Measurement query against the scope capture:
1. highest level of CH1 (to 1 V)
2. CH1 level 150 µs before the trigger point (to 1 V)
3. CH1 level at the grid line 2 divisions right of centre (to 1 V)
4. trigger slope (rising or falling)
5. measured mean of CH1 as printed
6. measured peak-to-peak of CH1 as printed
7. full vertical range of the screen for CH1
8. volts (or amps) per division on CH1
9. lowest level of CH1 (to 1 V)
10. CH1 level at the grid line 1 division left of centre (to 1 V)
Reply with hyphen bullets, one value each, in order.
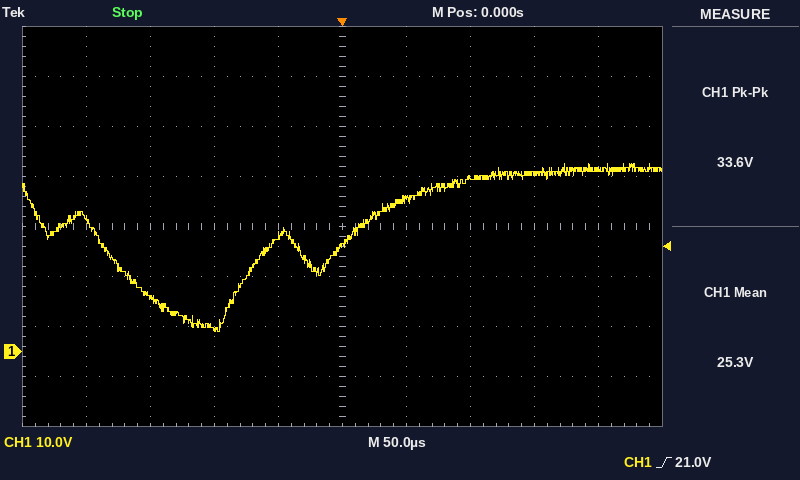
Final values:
- 38 V
- 11 V
- 35 V
- rising
- 25.3 V
- 33.6 V
- 80 V
- 10 V
- 4 V
- 23 V
